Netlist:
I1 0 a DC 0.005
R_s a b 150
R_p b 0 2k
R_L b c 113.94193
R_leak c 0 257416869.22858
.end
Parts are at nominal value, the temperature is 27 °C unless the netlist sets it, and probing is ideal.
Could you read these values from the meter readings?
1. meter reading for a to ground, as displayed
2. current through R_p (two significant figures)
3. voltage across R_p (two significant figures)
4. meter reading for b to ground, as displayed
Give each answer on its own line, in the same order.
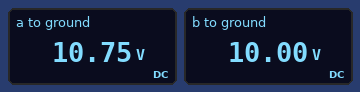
10.75 V
5.0 mA
10 V
10.00 V
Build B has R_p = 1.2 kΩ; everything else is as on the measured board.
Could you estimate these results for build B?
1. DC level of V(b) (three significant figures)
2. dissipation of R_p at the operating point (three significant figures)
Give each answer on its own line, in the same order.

6.00 V
30.0 mW
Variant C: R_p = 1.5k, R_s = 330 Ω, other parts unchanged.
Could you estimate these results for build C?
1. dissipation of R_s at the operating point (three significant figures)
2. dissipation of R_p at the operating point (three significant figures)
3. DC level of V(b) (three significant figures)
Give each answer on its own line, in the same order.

8.25 mW
37.5 mW
7.50 V
